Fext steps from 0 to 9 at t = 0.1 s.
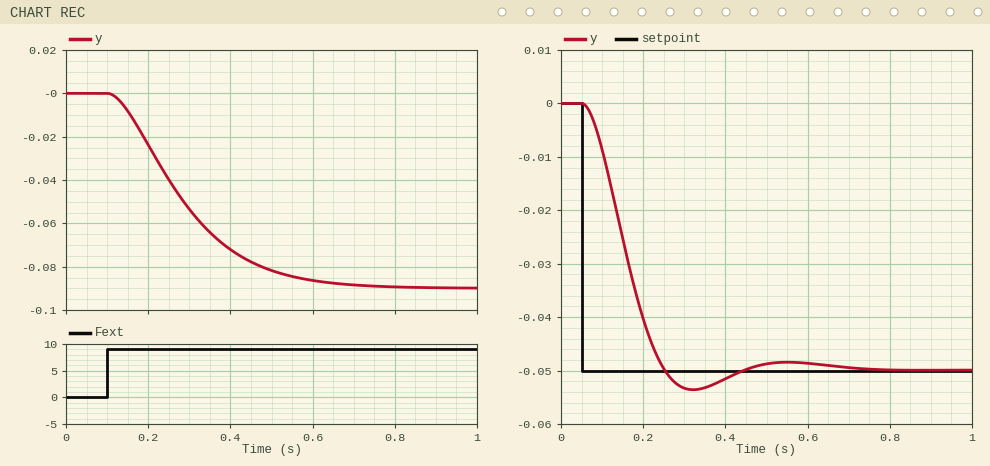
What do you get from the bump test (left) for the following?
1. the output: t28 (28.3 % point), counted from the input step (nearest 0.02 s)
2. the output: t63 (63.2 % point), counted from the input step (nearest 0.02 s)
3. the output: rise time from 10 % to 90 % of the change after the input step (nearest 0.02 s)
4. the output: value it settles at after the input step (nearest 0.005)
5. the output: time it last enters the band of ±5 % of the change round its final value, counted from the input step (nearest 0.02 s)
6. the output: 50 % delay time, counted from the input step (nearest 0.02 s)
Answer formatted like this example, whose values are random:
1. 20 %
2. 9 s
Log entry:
1. 0.10 s
2. 0.22 s
3. 0.34 s
4. -0.090
5. 0.48 s
6. 0.16 s
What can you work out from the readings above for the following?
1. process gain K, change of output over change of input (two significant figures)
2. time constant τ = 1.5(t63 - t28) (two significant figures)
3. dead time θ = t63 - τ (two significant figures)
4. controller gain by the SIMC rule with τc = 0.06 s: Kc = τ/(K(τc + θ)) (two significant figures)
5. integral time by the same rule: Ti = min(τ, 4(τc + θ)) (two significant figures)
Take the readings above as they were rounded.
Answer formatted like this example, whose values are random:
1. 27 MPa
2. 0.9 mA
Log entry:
1. -0.010
2. 0.18 s
3. 0.040 s
4. -180
5. 0.18 s
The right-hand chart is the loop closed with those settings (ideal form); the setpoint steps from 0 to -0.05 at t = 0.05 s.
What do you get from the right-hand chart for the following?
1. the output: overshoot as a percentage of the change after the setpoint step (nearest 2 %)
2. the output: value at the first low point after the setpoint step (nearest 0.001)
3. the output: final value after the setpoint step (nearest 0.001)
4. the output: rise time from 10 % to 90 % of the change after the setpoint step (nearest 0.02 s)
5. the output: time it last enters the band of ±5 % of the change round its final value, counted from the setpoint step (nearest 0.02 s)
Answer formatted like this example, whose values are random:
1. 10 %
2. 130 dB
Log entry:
1. 8 %
2. -0.054
3. -0.050
4. 0.14 s
5. 0.32 s
